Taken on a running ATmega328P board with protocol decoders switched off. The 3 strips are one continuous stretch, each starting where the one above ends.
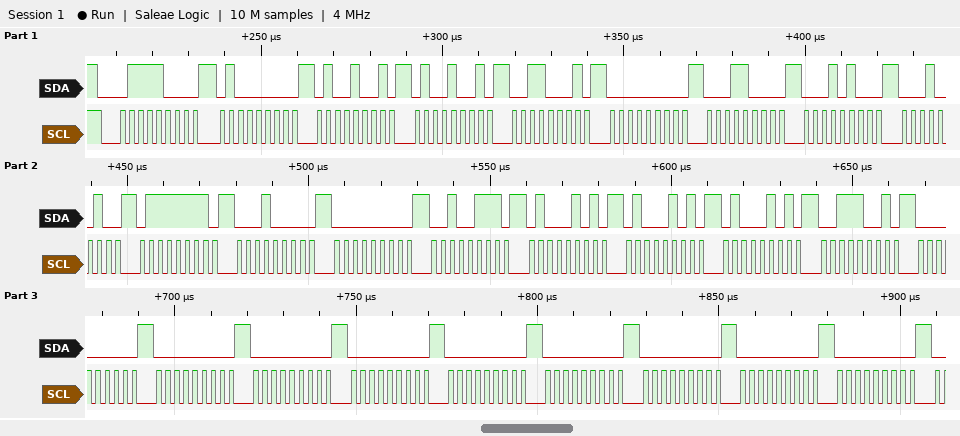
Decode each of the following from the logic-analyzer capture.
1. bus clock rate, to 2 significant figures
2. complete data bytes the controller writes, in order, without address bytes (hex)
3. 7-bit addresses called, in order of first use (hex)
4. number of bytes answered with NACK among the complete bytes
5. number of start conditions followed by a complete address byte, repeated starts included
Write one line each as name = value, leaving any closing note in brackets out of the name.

bus clock rate, to 2 significant figures = 400 kHz
complete data bytes the controller writes, in order, without address bytes = 40 49 49 31 00 18 14 12 7F 10 00 27 45 45 45 39 00 00 00 00 00 00 00 00 00
7-bit addresses called, in order of first use = 0x3C
number of bytes answered with NACK among the complete bytes = 0
number of start conditions followed by a complete address byte, repeated starts included = 1
